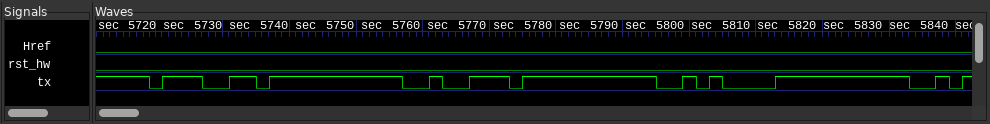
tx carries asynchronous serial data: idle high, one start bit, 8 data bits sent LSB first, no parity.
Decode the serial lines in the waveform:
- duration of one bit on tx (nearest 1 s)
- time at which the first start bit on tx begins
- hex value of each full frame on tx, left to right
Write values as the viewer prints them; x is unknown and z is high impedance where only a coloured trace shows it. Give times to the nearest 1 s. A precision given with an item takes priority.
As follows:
2 s
5719 s
67, 72, 0A
